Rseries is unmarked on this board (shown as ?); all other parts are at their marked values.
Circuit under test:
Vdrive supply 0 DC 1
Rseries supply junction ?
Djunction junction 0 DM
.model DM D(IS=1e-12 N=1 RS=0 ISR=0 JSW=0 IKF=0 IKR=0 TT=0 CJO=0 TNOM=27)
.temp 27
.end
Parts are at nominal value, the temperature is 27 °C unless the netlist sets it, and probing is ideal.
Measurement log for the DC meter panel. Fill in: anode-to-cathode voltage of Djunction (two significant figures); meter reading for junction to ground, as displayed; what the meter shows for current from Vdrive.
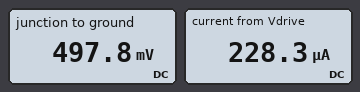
500 mV
497.8 mV
228.3 µA
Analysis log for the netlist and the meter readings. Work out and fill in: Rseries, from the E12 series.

2.2 kΩ
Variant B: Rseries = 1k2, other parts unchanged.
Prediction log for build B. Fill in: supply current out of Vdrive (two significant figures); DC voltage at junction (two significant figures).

410 µA
510 mV
